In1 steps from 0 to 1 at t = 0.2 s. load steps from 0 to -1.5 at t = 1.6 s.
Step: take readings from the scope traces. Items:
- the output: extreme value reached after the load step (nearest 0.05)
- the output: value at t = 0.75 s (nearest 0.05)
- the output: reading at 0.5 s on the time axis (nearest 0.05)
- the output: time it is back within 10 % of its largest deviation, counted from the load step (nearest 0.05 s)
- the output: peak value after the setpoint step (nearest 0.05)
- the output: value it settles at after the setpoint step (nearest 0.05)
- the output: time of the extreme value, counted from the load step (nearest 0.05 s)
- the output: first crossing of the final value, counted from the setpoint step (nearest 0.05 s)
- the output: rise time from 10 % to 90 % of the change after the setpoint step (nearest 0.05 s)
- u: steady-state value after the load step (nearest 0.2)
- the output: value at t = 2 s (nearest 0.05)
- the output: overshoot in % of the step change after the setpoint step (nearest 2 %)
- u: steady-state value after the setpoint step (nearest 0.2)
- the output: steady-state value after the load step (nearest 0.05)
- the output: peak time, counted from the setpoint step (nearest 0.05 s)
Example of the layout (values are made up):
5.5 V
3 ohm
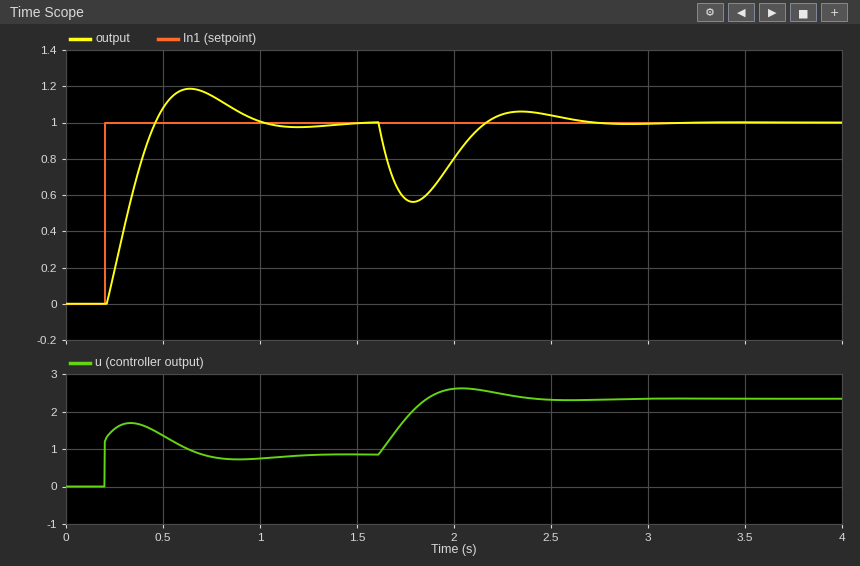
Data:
0.55
1.15
1.10
0.90 s
1.20
1.00
0.20 s
0.25 s
0.20 s
2.4
0.80
18 %
0.8
1.00
0.45 s
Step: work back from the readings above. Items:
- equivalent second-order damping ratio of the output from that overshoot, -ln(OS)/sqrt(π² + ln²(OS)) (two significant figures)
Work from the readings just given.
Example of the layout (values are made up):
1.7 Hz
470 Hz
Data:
0.48
